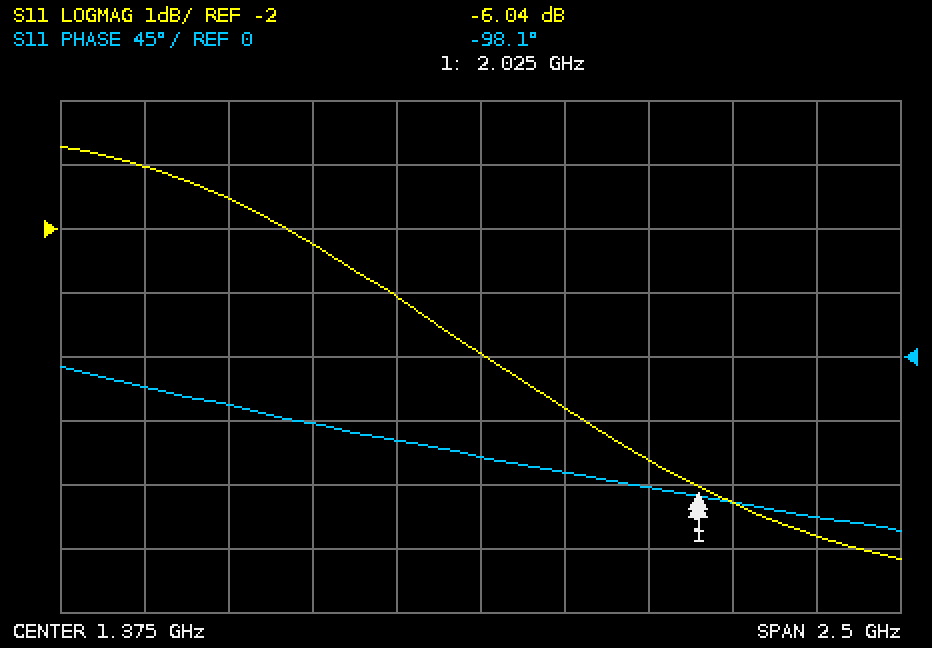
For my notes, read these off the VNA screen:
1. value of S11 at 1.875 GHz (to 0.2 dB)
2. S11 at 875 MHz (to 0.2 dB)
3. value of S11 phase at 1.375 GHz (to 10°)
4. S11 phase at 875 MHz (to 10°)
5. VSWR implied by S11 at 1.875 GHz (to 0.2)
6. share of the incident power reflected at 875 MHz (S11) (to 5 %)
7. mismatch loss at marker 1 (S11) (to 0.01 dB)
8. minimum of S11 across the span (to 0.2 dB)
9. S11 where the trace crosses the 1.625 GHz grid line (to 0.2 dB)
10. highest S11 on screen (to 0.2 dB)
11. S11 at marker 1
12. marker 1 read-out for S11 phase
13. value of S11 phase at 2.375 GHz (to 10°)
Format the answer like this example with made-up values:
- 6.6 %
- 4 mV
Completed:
- -5.6 dB
- -2.2 dB
- -70°
- -50°
- 3.2
- 60 %
- 1.24 dB
- -7.2 dB
- -4.8 dB
- -0.8 dB
- -6.04 dB
- -98.1°
- -110°
